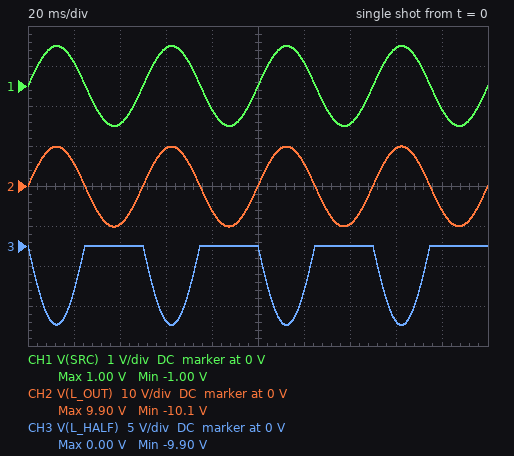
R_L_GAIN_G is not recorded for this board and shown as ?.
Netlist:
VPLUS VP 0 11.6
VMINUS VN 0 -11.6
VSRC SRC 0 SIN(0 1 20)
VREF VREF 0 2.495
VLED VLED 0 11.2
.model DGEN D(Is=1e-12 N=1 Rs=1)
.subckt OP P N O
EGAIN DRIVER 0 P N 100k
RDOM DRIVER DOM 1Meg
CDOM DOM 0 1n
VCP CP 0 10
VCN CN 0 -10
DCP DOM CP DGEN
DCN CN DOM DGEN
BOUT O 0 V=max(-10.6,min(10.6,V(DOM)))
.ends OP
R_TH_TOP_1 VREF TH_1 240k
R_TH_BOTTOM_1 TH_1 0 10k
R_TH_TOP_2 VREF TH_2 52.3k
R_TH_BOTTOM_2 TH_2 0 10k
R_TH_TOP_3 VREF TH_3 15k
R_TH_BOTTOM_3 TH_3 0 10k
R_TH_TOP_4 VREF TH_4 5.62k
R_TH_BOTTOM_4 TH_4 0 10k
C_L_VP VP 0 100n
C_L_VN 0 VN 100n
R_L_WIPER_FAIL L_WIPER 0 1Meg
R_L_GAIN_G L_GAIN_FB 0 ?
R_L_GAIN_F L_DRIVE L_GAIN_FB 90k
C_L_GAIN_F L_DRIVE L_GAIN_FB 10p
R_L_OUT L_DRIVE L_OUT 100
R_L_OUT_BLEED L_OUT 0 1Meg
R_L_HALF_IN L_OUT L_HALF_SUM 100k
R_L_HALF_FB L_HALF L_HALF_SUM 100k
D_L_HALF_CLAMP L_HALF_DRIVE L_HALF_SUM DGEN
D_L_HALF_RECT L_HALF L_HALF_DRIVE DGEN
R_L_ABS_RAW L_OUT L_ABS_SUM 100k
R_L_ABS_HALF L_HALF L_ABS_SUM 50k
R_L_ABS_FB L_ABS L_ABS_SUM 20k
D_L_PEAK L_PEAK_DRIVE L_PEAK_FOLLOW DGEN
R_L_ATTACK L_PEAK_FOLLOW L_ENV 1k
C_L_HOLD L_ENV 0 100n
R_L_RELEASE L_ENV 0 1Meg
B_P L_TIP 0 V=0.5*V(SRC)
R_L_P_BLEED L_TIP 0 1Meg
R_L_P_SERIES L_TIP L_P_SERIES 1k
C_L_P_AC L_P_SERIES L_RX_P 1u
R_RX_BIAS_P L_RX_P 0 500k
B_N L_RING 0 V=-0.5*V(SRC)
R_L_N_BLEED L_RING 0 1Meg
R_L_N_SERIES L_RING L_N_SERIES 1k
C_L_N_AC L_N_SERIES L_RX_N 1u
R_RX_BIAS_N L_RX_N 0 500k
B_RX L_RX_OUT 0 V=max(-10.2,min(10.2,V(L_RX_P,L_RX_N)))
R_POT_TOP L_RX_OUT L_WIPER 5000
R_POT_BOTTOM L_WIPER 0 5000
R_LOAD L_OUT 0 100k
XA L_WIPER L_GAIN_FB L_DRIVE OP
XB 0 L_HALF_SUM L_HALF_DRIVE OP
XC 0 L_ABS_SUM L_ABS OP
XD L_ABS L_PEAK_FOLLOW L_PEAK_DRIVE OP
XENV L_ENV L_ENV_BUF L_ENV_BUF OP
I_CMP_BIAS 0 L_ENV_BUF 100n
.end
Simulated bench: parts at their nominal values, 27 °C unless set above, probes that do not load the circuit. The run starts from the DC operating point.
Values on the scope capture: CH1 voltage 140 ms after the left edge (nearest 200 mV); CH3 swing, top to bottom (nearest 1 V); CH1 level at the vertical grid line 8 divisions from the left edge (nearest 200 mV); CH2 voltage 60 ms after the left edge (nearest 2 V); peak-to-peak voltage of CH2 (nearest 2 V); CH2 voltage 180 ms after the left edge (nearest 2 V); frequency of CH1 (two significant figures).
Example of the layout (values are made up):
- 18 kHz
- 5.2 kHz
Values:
- -1.0 V
- 10 V
- 1.0 V
- 10 V
- 20 V
- -6 V
- 20 Hz
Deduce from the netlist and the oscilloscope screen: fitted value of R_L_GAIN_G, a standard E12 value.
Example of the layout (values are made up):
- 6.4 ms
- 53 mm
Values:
- 4.7 kΩ
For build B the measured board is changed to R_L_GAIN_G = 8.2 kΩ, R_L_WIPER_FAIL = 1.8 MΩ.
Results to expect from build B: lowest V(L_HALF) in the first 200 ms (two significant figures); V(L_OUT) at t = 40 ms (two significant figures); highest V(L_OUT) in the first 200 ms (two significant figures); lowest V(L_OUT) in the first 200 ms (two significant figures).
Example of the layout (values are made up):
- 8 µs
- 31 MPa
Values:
- -5.9 V
- -5.7 V
- 5.9 V
- -6.0 V
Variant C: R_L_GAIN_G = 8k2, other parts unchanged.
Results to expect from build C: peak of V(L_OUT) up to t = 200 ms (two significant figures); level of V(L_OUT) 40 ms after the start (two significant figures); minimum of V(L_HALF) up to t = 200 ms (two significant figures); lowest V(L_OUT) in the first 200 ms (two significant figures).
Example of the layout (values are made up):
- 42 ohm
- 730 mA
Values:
- 5.9 V
- -5.7 V
- -5.9 V
- -6.0 V
